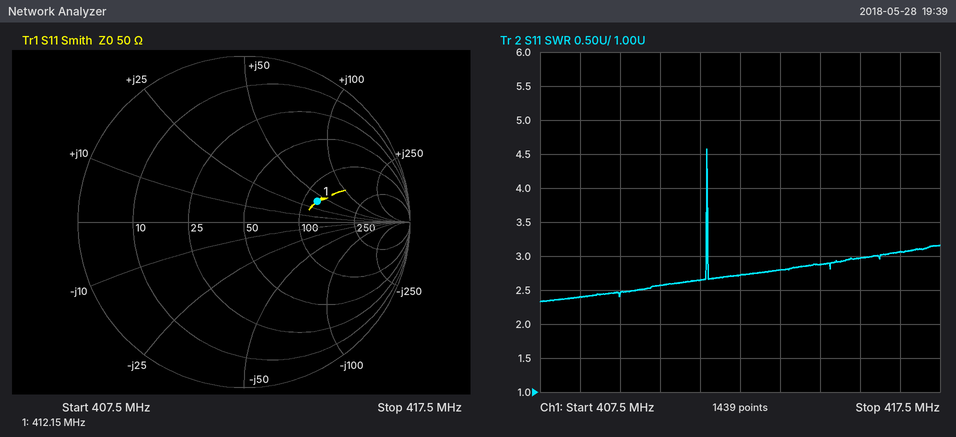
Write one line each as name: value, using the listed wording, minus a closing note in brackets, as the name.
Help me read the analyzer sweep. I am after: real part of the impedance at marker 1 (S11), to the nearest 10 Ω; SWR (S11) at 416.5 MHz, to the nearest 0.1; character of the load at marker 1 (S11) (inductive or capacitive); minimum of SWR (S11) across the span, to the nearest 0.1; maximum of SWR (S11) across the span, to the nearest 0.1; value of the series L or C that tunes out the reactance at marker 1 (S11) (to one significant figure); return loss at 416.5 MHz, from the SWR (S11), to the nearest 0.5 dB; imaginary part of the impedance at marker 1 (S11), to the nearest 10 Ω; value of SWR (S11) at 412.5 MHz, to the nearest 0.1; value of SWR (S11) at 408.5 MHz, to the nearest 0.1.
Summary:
real part of the impedance at marker 1 (S11), to the nearest 10 Ω: 120 Ω
SWR (S11) at 416.5 MHz, to the nearest 0.1: 3.1
character of the load at marker 1 (S11): inductive
minimum of SWR (S11) across the span, to the nearest 0.1: 2.3
maximum of SWR (S11) across the span, to the nearest 0.1: 4.6
value of the series L or C that tunes out the reactance at marker 1 (S11): 10 pF
return loss at 416.5 MHz, from the SWR (S11), to the nearest 0.5 dB: 6.0 dB
imaginary part of the impedance at marker 1 (S11), to the nearest 10 Ω: +40 Ω
value of SWR (S11) at 412.5 MHz, to the nearest 0.1: 2.7
value of SWR (S11) at 408.5 MHz, to the nearest 0.1: 2.4
